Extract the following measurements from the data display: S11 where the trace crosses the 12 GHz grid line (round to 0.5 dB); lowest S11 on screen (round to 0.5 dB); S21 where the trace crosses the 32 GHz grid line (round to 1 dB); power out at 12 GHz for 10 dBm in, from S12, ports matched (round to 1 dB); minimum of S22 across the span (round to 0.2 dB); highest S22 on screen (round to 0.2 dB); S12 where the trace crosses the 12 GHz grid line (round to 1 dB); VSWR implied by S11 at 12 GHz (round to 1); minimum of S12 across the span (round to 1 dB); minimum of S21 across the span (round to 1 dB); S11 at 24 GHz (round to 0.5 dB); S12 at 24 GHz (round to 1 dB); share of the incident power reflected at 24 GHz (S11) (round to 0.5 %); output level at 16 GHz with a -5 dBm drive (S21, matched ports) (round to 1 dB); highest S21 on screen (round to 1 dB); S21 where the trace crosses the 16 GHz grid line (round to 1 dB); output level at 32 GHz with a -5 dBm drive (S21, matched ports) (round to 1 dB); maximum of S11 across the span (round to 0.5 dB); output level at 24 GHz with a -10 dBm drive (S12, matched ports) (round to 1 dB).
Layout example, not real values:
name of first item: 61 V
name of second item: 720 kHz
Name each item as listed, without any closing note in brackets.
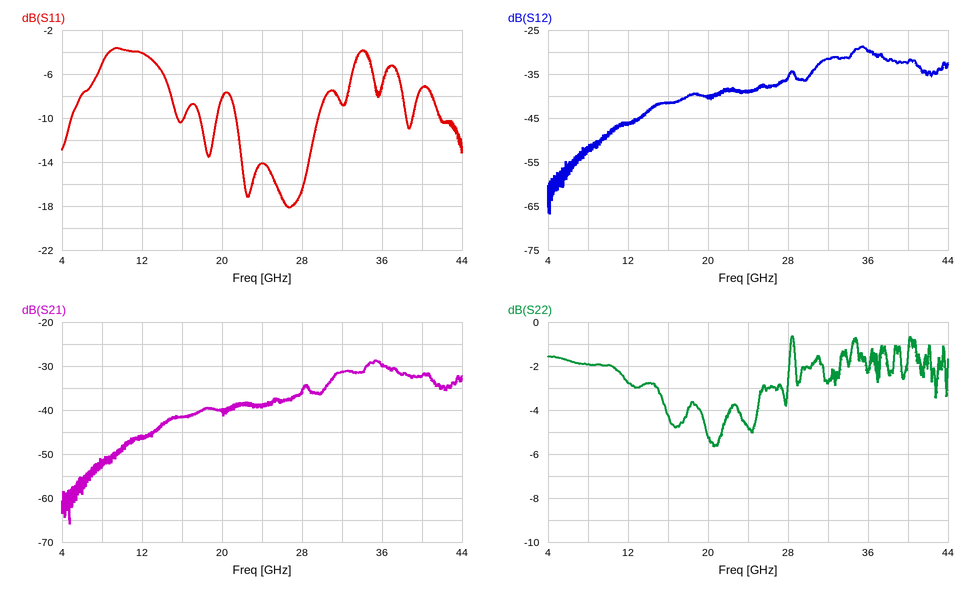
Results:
S11 where the trace crosses the 12 GHz grid line: -4.0 dB
lowest S11 on screen: -18.0 dB
S21 where the trace crosses the 32 GHz grid line: -31 dB
power out at 12 GHz for 10 dBm in, from S12, ports matched: -36 dBm
minimum of S22 across the span: -5.6 dB
highest S22 on screen: -0.6 dB
S12 where the trace crosses the 12 GHz grid line: -46 dB
VSWR implied by S11 at 12 GHz: 4
minimum of S12 across the span: -67 dB
minimum of S21 across the span: -66 dB
S11 at 24 GHz: -14.0 dB
S12 at 24 GHz: -39 dB
share of the incident power reflected at 24 GHz (S11): 4.0 %
output level at 16 GHz with a -5 dBm drive (S21, matched ports): -47 dBm
highest S21 on screen: -29 dB
S21 where the trace crosses the 16 GHz grid line: -42 dB
output level at 32 GHz with a -5 dBm drive (S21, matched ports): -36 dBm
maximum of S11 across the span: -3.5 dB
output level at 24 GHz with a -10 dBm drive (S12, matched ports): -49 dBm
